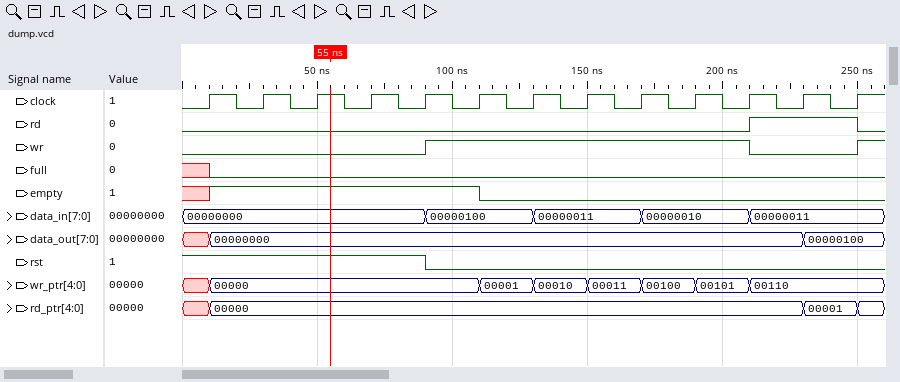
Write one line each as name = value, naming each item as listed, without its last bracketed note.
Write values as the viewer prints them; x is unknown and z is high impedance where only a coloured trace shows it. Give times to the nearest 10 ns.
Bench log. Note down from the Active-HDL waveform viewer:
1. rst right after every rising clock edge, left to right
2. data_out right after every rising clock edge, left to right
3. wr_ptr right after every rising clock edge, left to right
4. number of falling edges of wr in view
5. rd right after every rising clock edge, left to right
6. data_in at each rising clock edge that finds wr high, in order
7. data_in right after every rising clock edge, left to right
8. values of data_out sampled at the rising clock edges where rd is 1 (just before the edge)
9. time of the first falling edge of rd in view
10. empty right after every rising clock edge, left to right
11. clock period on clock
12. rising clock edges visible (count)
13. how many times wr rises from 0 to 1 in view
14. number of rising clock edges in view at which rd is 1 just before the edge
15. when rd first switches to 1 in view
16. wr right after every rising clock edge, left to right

rst right after every rising clock edge, left to right = 1 1 1 1 0 0 0 0 0 0 0 0 0
data_out right after every rising clock edge, left to right = 00000000, 00000000, 00000000, 00000000, 00000000, 00000000, 00000000, 00000000, 00000000, 00000000, 00000000, 00000100, 00000100
wr_ptr right after every rising clock edge, left to right = 00000, 00000, 00000, 00000, 00000, 00001, 00010, 00011, 00100, 00101, 00110, 00110, 00110
number of falling edges of wr in view = 1
rd right after every rising clock edge, left to right = 0 0 0 0 0 0 0 0 0 0 1 1 0
data_in at each rising clock edge that finds wr high, in order = 00000100, 00000100, 00000011, 00000011, 00000010, 00000010
data_in right after every rising clock edge, left to right = 00000000, 00000000, 00000000, 00000000, 00000100, 00000100, 00000011, 00000011, 00000010, 00000010, 00000011, 00000011, 00000011
values of data_out sampled at the rising clock edges where rd is 1 = 00000000, 00000100
time of the first falling edge of rd in view = 250 ns
empty right after every rising clock edge, left to right = 1 1 1 1 1 0 0 0 0 0 0 0 0
clock period on clock = 20 ns
rising clock edges visible = 13
how many times wr rises from 0 to 1 in view = 2
number of rising clock edges in view at which rd is 1 just before the edge = 2
when rd first switches to 1 in view = 210 ns
wr right after every rising clock edge, left to right = 0 0 0 0 1 1 1 1 1 1 0 0 1
